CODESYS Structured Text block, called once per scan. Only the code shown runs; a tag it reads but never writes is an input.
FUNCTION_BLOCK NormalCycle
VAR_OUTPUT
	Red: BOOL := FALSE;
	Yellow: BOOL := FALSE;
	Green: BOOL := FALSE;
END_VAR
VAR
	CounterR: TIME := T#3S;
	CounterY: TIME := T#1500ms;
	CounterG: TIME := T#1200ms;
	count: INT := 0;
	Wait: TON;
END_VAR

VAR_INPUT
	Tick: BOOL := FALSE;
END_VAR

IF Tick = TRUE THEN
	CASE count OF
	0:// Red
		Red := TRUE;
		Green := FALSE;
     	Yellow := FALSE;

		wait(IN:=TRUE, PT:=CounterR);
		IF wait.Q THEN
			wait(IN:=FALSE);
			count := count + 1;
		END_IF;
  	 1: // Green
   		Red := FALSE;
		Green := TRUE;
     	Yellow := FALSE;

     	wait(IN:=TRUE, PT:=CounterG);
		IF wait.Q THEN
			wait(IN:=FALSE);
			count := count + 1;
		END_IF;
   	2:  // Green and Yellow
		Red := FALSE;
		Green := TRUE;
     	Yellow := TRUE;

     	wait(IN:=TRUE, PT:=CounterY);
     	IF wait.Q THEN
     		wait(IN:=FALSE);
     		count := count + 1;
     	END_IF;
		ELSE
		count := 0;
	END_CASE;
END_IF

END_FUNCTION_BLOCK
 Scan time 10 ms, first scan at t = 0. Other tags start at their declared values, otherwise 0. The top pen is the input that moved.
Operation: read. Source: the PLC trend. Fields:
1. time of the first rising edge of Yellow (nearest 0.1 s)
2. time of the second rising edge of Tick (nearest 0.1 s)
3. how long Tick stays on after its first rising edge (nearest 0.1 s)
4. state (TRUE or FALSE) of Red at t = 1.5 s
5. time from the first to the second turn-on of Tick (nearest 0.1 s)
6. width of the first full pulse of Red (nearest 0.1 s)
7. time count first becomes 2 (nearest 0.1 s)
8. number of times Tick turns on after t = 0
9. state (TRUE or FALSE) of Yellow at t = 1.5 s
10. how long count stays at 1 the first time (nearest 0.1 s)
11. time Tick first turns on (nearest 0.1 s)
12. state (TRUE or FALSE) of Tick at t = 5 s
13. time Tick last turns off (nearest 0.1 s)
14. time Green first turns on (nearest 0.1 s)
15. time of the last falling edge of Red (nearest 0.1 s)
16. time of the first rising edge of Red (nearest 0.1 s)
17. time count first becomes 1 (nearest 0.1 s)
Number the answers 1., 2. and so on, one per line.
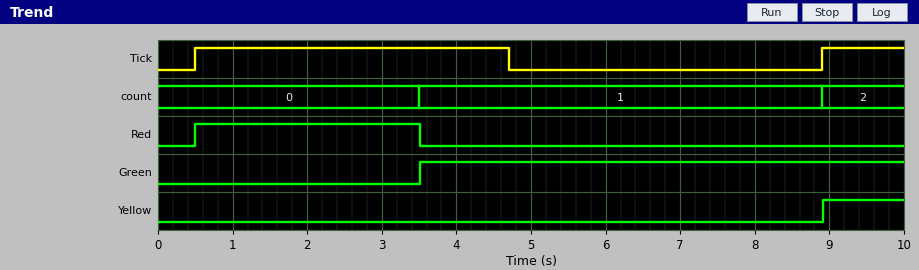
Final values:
1. 8.9 s
2. 8.9 s
3. 4.2 s
4. TRUE
5. 8.4 s
6. 3.0 s
7. 8.9 s
8. 2
9. FALSE
10. 5.4 s
11. 0.5 s
12. FALSE
13. 4.7 s
14. 3.5 s
15. 3.5 s
16. 0.5 s
17. 3.5 s
